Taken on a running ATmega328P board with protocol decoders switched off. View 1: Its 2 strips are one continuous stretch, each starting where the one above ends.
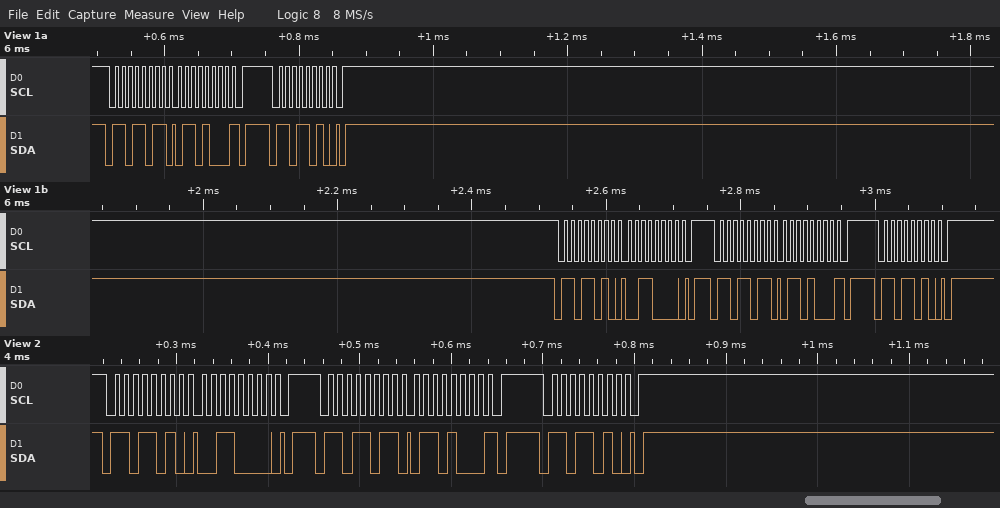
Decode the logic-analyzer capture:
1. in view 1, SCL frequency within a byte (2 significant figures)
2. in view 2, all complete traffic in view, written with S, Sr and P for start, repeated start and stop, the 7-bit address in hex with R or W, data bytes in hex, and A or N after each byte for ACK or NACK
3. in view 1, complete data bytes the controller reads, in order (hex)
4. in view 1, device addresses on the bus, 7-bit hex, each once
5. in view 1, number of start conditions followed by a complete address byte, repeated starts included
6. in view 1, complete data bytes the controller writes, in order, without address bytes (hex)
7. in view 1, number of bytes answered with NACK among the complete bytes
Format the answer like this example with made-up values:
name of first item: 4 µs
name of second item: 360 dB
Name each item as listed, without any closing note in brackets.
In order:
in view 1, SCL frequency within a byte: 100 kHz
in view 2, all complete traffic in view, written with S, Sr and P for start, repeated start and stop, the 7-bit address in hex with R or W, data bytes in hex, and A or N after each byte for ACK or NACK: S 6DW A 30 A P S 6DR A 68 N P S 6DW A P
in view 1, complete data bytes the controller reads, in order: 68 68
in view 1, device addresses on the bus, 7-bit hex, each once: 0x6D
in view 1, number of start conditions followed by a complete address byte, repeated starts included: 5
in view 1, complete data bytes the controller writes, in order, without address bytes: 30
in view 1, number of bytes answered with NACK among the complete bytes: 2
